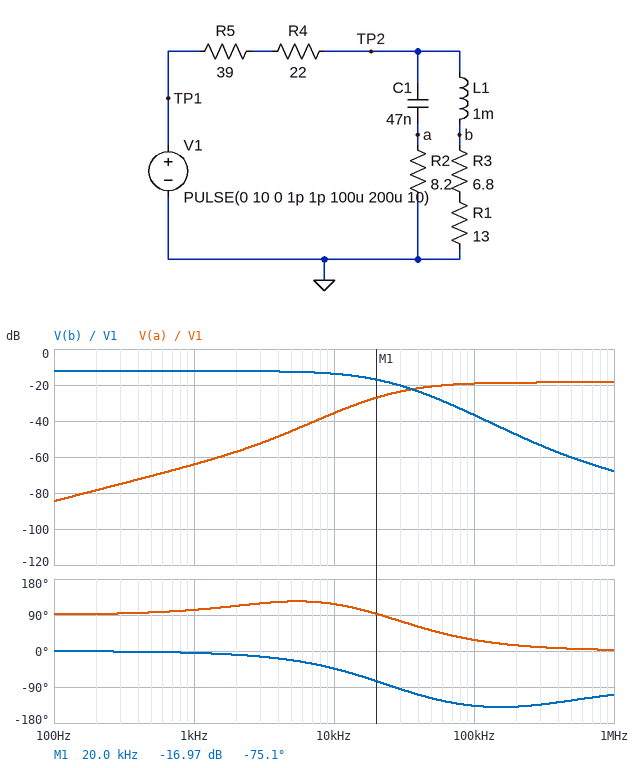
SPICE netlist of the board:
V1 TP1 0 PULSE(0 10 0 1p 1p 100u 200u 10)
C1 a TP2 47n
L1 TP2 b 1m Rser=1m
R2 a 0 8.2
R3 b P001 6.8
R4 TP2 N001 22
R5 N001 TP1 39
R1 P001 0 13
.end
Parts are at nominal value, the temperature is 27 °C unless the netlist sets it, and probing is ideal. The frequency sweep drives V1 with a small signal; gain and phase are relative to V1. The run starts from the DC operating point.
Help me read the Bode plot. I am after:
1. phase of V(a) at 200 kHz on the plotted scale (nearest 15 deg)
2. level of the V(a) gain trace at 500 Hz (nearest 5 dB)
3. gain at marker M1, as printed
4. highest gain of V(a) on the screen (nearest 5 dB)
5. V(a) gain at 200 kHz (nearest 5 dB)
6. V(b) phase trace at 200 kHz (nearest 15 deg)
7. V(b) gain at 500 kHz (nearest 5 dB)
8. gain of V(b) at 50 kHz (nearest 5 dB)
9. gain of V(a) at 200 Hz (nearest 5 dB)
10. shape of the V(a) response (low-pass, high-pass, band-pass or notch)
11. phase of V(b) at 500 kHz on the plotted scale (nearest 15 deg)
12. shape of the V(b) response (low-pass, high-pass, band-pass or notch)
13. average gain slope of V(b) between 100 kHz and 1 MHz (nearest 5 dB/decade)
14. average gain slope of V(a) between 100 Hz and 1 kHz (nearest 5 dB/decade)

15 deg
-70 dB
-16.97 dB
-20 dB
-20 dB
-135 deg
-60 dB
-25 dB
-80 dB
high-pass
-120 deg
low-pass
-30 dB/decade
20 dB/decade
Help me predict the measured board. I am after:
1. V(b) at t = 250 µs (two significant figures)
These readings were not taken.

2.4 V
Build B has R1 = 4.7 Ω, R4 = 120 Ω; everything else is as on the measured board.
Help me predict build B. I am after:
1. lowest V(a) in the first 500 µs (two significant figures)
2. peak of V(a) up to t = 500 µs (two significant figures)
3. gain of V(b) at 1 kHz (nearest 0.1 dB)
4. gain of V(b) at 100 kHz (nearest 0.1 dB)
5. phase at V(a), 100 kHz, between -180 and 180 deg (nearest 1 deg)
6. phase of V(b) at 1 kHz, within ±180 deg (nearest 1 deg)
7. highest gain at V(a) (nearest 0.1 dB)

-490 mV
490 mV
-23.4 dB
-48.1 dB
13 deg
-2 deg
-24.9 dB
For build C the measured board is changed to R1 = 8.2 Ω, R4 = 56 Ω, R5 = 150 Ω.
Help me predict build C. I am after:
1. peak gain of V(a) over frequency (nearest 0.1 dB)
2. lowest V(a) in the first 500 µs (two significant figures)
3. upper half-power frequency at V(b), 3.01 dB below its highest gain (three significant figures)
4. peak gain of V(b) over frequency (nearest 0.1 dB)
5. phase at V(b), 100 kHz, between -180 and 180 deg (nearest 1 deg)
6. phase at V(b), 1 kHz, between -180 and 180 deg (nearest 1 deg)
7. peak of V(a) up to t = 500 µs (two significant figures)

-25.8 dB
-380 mV
28.0 kHz
-20.9 dB
-155 deg
-2 deg
380 mV
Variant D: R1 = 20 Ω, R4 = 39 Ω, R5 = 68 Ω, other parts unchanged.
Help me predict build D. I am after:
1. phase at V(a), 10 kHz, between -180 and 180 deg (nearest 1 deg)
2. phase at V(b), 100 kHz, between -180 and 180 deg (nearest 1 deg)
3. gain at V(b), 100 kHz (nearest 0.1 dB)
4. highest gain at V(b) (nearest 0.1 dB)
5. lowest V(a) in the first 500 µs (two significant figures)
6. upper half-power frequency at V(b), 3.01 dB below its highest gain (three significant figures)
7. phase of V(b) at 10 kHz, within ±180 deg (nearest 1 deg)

123 deg
-146 deg
-37.8 dB
-14.0 dB
-710 mV
25.4 kHz
-32 deg
